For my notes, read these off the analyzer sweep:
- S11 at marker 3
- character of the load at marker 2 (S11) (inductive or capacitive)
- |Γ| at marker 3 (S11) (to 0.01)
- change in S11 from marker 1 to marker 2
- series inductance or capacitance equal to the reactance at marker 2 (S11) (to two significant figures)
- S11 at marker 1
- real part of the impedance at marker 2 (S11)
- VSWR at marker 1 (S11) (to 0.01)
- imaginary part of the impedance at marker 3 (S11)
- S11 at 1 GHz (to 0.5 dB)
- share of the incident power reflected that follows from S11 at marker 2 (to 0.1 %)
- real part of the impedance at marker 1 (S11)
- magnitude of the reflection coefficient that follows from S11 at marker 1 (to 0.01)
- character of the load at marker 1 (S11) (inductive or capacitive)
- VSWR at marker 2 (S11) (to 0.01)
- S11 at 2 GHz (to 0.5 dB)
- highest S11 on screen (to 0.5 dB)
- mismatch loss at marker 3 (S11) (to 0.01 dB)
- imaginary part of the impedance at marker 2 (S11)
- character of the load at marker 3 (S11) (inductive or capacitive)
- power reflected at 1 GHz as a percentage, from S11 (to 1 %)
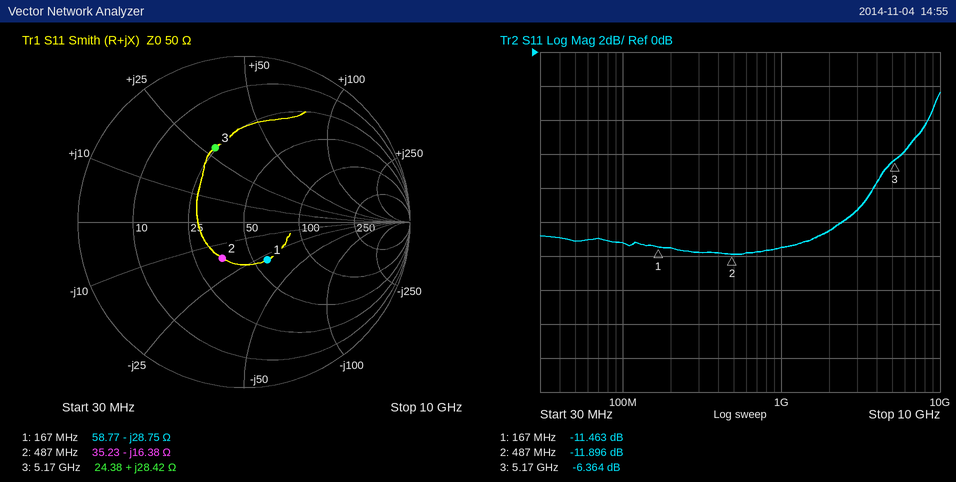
-6.364 dB
capacitive
0.48
-0.433 dB
20 pF
-11.463 dB
35.23 Ω
1.73
+28.42 Ω
-11.5 dB
6.5 %
58.77 Ω
0.27
capacitive
1.68
-10.5 dB
-2.5 dB
1.14 dB
-16.38 Ω
inductive
7 %
